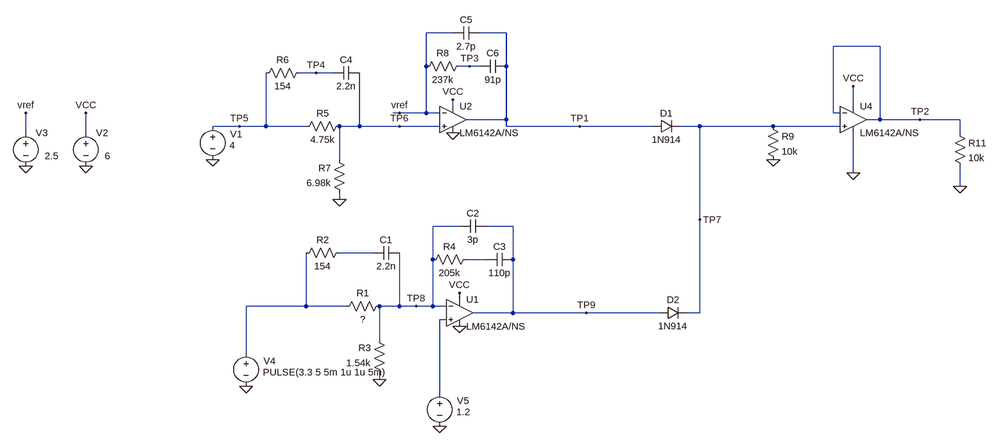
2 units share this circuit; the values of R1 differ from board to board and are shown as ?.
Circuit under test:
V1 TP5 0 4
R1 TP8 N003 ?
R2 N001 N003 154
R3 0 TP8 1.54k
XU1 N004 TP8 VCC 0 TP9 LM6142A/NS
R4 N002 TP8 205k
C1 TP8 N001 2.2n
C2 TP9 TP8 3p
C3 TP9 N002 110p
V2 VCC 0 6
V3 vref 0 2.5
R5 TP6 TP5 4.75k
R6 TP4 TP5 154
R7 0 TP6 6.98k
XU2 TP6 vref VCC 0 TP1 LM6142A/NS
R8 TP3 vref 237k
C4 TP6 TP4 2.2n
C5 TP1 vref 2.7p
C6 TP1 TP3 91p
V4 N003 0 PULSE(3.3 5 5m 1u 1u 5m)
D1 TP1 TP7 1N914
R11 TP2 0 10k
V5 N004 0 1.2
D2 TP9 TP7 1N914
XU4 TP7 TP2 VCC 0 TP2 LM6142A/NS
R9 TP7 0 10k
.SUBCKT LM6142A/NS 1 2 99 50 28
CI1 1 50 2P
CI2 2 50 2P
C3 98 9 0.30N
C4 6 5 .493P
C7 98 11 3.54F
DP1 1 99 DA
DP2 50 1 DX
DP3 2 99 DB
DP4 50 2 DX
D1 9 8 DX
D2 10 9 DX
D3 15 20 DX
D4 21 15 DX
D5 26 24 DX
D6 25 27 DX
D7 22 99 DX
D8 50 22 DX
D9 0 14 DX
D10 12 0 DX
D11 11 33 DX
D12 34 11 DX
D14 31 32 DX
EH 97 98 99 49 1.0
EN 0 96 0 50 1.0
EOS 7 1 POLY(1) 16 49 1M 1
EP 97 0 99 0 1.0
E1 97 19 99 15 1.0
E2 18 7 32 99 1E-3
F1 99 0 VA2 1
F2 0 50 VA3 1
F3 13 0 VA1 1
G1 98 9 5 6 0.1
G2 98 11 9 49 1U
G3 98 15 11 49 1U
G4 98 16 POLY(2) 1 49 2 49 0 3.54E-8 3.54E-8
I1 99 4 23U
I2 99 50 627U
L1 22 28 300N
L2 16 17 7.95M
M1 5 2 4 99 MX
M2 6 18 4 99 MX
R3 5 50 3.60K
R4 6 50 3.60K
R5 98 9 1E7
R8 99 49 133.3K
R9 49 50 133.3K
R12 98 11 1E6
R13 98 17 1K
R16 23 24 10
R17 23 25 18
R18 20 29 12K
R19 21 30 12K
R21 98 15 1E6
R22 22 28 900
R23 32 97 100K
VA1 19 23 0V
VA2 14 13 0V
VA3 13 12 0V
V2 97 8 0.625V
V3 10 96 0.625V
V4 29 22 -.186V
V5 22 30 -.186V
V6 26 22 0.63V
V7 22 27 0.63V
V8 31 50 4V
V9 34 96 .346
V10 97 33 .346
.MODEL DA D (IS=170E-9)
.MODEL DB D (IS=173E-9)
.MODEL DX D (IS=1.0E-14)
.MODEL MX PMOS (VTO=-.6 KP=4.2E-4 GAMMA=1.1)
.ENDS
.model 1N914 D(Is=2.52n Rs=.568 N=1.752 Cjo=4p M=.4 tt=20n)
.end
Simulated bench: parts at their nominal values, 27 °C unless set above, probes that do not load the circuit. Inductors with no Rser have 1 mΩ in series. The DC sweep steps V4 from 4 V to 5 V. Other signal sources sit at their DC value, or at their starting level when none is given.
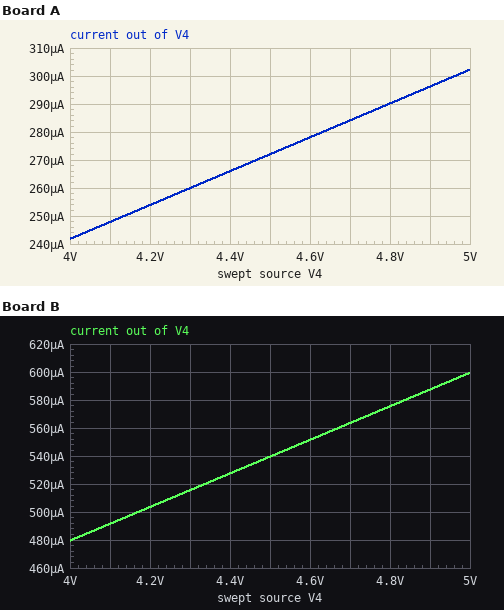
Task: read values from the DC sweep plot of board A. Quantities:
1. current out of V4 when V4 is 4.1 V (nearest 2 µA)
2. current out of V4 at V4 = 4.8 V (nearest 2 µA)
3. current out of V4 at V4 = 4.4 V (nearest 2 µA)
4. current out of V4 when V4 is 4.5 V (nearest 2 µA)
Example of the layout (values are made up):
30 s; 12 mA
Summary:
248 µA; 290 µA; 266 µA; 272 µA
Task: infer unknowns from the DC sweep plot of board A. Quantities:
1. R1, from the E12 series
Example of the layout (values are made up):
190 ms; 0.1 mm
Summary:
15 kΩ
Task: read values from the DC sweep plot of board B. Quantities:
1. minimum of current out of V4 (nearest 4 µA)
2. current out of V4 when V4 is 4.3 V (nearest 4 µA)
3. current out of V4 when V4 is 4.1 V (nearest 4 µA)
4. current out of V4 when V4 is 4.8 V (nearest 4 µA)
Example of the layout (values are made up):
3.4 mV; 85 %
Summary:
480 µA; 516 µA; 492 µA; 576 µA
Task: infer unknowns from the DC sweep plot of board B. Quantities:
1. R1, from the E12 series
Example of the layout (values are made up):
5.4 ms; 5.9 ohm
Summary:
6.8 kΩ
